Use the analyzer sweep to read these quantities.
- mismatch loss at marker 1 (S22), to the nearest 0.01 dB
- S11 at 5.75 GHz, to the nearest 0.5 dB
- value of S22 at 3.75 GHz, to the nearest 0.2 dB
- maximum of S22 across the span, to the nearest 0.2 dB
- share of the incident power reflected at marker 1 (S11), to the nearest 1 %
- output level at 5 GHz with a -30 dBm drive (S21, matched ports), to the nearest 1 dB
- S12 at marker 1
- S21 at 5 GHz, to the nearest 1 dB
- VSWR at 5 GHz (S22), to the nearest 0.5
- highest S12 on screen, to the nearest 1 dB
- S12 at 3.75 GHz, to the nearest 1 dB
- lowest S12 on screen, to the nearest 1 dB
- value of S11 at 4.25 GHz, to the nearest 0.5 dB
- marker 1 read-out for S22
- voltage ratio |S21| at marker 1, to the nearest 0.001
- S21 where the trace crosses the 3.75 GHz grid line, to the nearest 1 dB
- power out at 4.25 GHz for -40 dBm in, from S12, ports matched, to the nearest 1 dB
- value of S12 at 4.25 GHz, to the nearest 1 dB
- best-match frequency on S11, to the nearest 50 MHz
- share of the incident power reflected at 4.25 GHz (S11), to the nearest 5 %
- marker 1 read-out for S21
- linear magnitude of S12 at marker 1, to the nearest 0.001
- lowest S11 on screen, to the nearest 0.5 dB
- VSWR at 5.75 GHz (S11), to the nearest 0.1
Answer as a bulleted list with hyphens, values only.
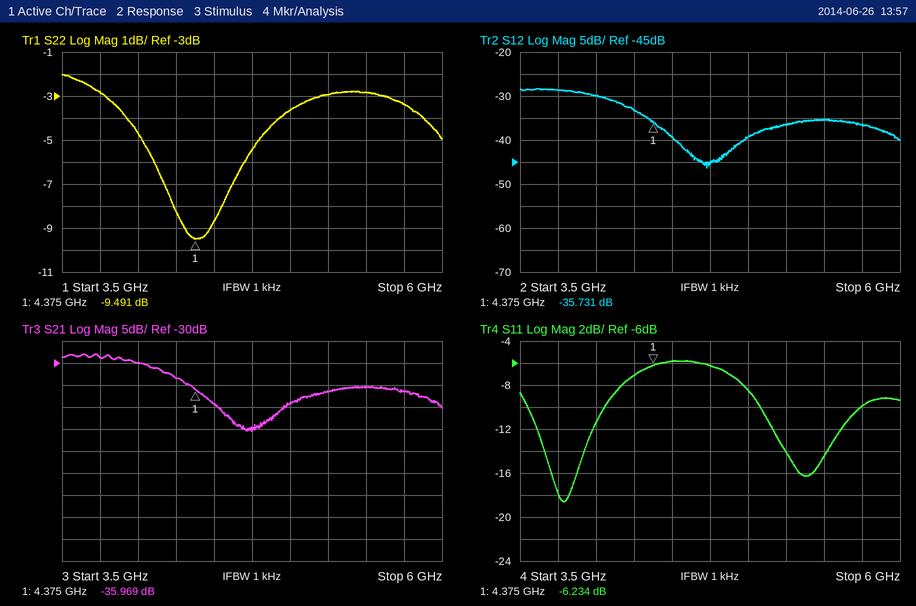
- 0.52 dB
- -10.0 dB
- -2.8 dB
- -2.0 dB
- 24 %
- -69 dBm
- -35.731 dB
- -39 dB
- 5.0
- -28 dB
- -29 dB
- -46 dB
- -7.0 dB
- -9.491 dB
- 0.016
- -29 dB
- -73 dBm
- -33 dB
- 3.80 GHz
- 20 %
- -35.969 dB
- 0.016
- -18.5 dB
- 1.9
